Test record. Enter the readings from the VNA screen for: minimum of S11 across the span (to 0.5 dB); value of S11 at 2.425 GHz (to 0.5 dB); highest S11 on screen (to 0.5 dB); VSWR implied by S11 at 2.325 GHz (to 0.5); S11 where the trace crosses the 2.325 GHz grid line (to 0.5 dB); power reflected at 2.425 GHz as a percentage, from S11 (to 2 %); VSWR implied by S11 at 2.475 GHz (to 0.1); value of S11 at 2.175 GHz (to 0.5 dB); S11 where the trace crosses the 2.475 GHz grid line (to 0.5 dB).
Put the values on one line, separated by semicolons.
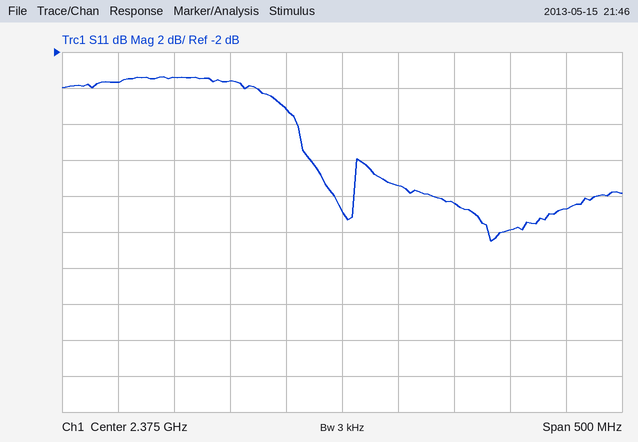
-12.5 dB; -9.5 dB; -3.5 dB; 3.5; -5.0 dB; 12 %; 1.9; -3.5 dB; -10.5 dB
